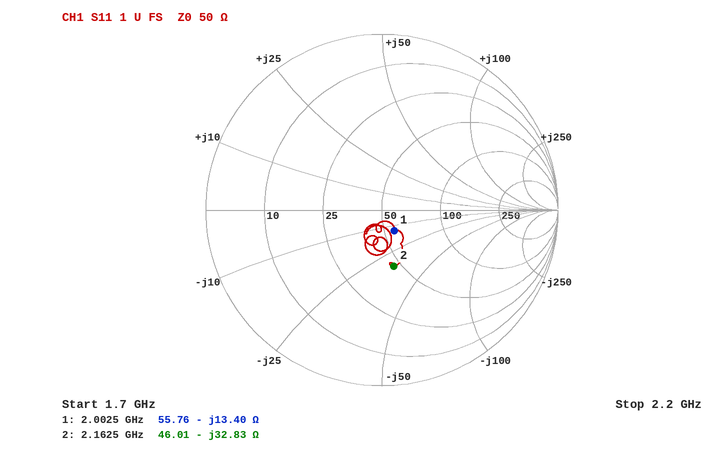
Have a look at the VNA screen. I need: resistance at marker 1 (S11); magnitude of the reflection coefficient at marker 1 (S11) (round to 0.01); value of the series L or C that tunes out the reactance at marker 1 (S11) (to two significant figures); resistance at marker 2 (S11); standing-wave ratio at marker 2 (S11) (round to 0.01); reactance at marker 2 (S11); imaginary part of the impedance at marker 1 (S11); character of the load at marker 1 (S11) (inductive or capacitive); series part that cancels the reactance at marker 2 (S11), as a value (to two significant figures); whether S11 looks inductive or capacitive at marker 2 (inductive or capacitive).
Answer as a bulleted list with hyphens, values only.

- 55.76 Ω
- 0.14
- 1.1 nH
- 46.01 Ω
- 1.97
- -32.83 Ω
- -13.40 Ω
- capacitive
- 2.4 nH
- capacitive
